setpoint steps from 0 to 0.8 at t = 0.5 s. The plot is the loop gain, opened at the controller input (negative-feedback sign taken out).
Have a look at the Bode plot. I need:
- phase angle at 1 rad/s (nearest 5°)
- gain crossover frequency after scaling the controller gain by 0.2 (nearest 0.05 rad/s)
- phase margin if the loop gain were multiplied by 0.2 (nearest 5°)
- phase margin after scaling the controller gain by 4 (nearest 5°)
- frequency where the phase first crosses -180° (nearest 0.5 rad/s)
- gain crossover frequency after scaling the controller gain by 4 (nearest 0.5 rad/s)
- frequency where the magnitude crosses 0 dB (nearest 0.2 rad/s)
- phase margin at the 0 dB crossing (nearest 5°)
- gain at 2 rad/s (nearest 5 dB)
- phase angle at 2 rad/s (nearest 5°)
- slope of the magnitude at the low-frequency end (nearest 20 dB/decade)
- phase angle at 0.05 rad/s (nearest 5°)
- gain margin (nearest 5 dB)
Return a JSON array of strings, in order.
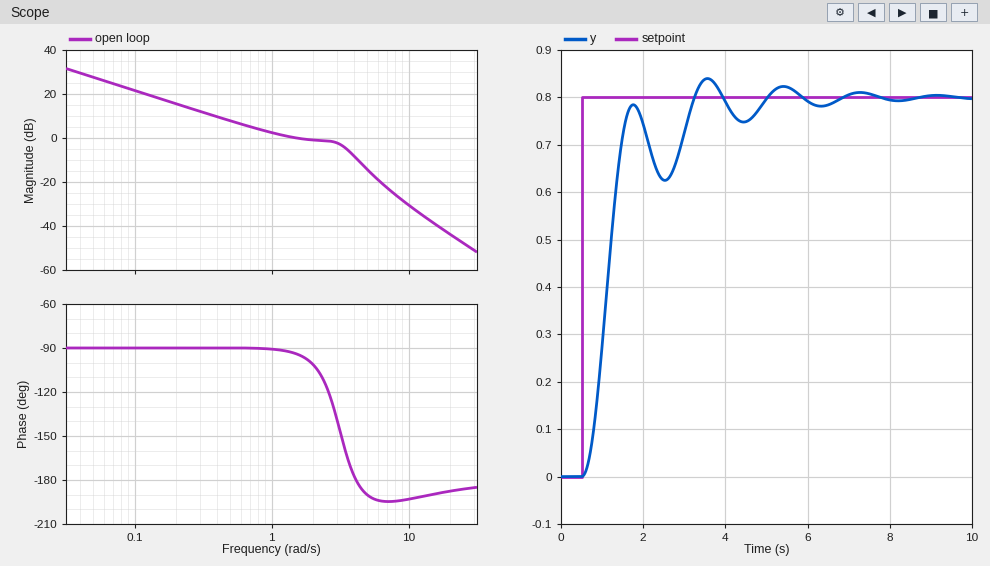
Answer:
["-90°", "0.25 rad/s", "90°", "-5°", "4.0 rad/s", "4.5 rad/s", "1.6 rad/s", "85°", "0 dB", "-100°", "-20 dB/decade", "-90°", "10 dB"]
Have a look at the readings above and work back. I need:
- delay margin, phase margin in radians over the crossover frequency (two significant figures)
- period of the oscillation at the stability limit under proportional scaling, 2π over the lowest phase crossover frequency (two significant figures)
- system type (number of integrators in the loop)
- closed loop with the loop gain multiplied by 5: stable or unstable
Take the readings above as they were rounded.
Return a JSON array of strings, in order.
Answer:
["0.93 s", "1.6 s", "1", "unstable"]
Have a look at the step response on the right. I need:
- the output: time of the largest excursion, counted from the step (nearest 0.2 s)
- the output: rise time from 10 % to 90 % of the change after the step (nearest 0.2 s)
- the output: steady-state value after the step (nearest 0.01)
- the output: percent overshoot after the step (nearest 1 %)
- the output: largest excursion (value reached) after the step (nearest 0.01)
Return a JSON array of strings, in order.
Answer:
["3.0 s", "0.8 s", "0.80", "5 %", "0.84"]
